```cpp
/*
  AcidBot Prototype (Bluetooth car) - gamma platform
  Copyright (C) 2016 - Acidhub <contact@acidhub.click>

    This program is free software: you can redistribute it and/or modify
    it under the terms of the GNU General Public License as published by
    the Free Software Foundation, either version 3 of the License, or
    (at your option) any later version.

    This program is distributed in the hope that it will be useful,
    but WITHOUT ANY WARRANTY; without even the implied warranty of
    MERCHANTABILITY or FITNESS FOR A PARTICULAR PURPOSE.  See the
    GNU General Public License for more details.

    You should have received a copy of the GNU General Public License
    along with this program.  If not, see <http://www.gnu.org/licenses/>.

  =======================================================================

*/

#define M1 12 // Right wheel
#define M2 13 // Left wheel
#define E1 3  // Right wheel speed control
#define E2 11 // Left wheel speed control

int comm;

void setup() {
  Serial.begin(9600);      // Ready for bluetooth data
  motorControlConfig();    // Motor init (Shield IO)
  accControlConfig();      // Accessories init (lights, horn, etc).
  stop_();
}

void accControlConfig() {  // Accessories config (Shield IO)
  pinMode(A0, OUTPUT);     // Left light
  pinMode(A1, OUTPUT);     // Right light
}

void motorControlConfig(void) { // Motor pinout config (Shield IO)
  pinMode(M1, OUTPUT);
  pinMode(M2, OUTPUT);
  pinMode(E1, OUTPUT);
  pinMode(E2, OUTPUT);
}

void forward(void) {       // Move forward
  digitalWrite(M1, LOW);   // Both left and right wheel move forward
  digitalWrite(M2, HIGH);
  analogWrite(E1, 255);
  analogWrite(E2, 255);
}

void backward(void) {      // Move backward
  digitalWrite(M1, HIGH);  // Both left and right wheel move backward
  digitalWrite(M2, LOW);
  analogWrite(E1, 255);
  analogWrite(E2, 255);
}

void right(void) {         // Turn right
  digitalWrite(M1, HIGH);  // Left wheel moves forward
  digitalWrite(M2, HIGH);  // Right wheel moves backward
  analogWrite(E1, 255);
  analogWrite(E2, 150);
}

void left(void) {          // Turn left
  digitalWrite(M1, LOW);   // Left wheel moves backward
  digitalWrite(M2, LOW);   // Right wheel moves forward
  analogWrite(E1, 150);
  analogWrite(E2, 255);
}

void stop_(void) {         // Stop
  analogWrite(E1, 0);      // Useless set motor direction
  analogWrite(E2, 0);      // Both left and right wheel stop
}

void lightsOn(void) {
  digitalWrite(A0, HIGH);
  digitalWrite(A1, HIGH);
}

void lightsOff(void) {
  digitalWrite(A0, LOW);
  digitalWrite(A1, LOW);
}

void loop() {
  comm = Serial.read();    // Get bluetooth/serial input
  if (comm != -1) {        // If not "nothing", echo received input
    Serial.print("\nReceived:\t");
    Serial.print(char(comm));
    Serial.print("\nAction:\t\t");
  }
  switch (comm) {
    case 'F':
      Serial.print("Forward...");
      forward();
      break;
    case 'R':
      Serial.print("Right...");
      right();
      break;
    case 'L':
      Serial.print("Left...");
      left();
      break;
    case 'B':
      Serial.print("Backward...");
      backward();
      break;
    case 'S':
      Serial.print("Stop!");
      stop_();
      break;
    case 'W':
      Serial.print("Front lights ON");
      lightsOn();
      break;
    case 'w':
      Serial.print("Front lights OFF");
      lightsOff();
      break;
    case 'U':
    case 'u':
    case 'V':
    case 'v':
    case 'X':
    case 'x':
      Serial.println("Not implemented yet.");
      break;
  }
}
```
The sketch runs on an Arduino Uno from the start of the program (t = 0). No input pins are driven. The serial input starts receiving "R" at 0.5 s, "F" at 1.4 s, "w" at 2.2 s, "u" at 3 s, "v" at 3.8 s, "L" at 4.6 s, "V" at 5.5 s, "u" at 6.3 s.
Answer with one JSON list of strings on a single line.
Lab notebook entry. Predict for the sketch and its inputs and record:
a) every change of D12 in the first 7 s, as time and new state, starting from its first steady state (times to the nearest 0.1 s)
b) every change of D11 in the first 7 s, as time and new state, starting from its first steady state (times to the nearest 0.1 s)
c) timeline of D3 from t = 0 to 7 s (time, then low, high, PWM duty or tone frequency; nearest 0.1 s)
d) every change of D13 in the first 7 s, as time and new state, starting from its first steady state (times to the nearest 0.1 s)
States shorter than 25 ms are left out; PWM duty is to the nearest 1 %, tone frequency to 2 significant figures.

["0 s low; 0.5 s high; 1.4 s low", "0 s low; 0.5 s PWM 59 %; 1.4 s high", "0 s low; 0.5 s high; 4.6 s PWM 59 %", "0 s low; 0.5 s high; 4.6 s low"]
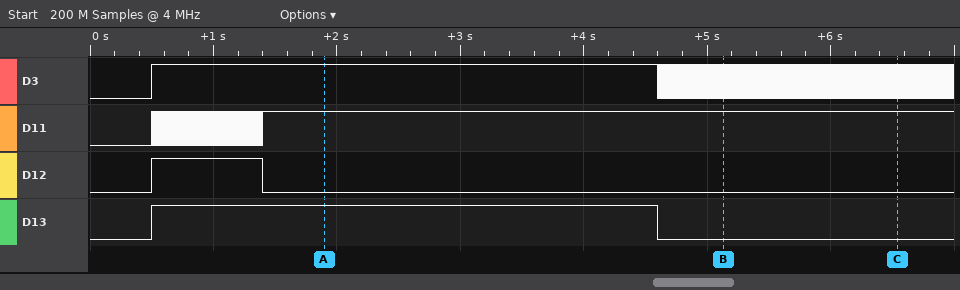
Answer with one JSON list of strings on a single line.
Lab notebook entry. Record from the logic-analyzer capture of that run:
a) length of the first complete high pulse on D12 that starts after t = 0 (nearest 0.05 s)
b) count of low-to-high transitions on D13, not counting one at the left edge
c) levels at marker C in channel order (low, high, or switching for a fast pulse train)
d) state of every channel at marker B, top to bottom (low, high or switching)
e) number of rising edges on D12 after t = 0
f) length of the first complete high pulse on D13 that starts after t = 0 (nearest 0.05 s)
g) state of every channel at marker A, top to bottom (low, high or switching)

["0.90 s", "1", "D3 switching, D11 high, D12 low, D13 low", "D3 switching, D11 high, D12 low, D13 low", "1", "4.10 s", "D3 high, D11 high, D12 low, D13 high"]
